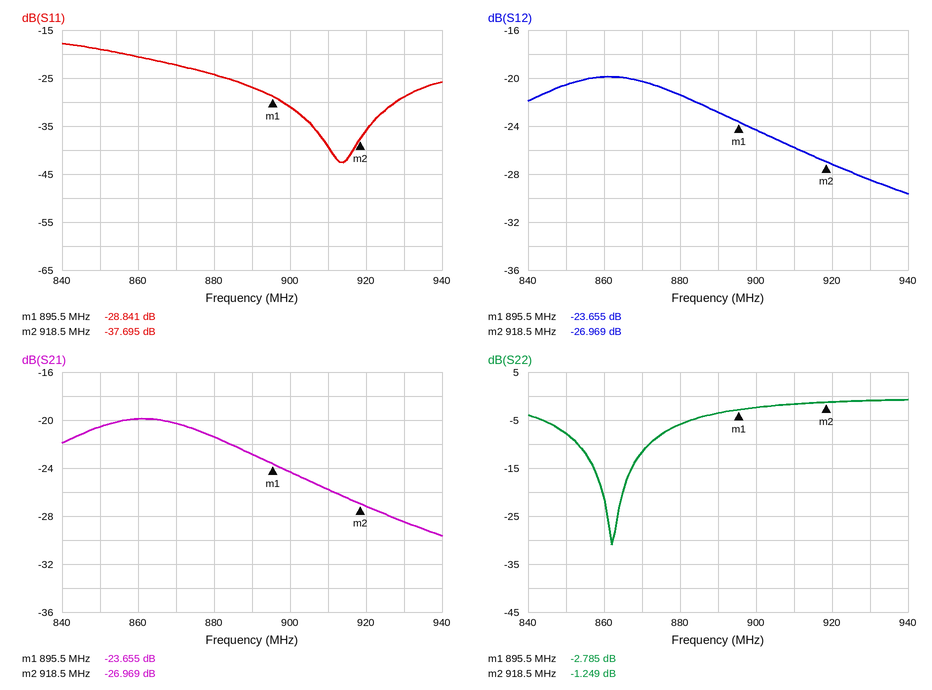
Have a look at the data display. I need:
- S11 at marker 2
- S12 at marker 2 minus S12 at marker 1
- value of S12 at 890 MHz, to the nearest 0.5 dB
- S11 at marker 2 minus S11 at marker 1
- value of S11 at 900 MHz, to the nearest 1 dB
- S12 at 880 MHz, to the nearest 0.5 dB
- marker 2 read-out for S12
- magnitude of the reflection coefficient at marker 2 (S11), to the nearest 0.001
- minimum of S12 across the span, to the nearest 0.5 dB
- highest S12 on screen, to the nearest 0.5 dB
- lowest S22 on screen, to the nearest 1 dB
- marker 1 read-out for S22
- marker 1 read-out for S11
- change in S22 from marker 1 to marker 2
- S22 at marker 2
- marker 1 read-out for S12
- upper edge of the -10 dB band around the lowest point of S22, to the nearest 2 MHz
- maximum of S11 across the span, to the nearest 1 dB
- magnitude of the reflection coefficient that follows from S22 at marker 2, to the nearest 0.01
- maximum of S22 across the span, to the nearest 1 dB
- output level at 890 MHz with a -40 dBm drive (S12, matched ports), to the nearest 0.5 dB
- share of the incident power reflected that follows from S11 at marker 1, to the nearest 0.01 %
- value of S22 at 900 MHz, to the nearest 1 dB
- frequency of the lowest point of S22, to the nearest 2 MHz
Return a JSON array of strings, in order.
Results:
["-37.695 dB", "-3.314 dB", "-23.0 dB", "-8.854 dB", "-31 dB", "-21.5 dB", "-26.969 dB", "0.013", "-29.5 dB", "-20.0 dB", "-31 dB", "-2.785 dB", "-28.841 dB", "1.536 dB", "-1.249 dB", "-23.655 dB", "872 MHz", "-18 dB", "0.87", "-1 dB", "-63.0 dBm", "0.13 %", "-2 dB", "862 MHz"]
